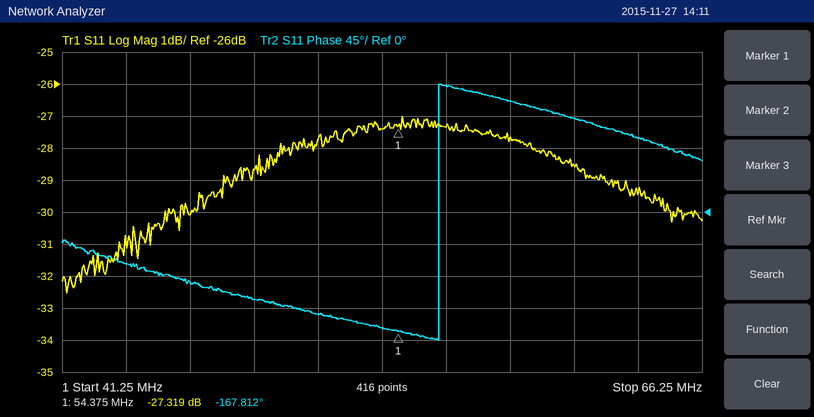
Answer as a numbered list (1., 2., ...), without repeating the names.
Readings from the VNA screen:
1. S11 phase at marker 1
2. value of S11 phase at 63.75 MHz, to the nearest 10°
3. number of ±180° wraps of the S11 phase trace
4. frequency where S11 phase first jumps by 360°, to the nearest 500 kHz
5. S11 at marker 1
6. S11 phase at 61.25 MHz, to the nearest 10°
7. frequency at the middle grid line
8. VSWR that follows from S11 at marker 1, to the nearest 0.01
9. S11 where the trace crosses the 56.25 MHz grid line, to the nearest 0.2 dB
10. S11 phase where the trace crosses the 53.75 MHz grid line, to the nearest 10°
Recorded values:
1. -167.812°
2. 100°
3. 1
4. 56.0 MHz
5. -27.319 dB
6. 130°
7. 53.75 MHz
8. 1.09
9. -27.4 dB
10. -160°
